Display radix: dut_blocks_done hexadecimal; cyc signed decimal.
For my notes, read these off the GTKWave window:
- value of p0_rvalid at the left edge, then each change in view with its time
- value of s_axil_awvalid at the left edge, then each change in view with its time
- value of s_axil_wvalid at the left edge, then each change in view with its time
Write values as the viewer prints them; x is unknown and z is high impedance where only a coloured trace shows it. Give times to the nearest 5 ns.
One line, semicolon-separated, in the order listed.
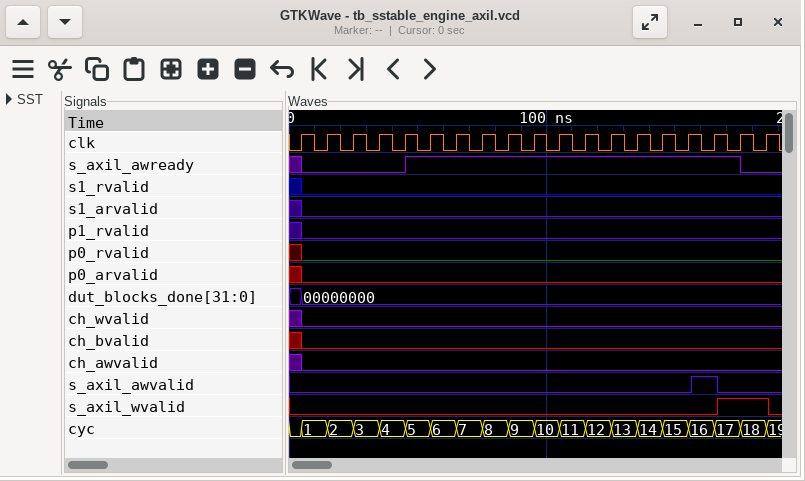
x, 0 at 5 ns; 0, 1 at 155 ns, 0 at 165 ns; 0, 1 at 165 ns, 0 at 185 ns
